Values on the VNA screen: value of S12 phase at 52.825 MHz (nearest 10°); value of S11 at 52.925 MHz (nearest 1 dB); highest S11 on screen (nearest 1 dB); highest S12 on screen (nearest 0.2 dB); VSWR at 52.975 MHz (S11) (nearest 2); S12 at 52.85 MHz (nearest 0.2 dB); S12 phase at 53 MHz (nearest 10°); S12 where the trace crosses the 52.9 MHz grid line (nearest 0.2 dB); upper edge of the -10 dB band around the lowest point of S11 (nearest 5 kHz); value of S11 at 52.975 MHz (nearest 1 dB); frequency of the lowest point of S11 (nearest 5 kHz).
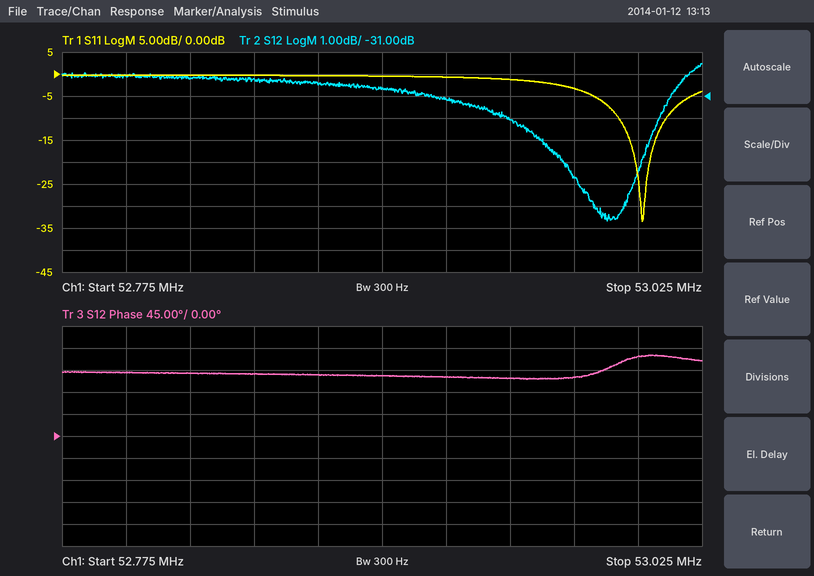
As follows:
130°
-1 dB
0 dB
-29.6 dB
6
-30.2 dB
160°
-30.6 dB
53.010 MHz
-3 dB
53.000 MHz
